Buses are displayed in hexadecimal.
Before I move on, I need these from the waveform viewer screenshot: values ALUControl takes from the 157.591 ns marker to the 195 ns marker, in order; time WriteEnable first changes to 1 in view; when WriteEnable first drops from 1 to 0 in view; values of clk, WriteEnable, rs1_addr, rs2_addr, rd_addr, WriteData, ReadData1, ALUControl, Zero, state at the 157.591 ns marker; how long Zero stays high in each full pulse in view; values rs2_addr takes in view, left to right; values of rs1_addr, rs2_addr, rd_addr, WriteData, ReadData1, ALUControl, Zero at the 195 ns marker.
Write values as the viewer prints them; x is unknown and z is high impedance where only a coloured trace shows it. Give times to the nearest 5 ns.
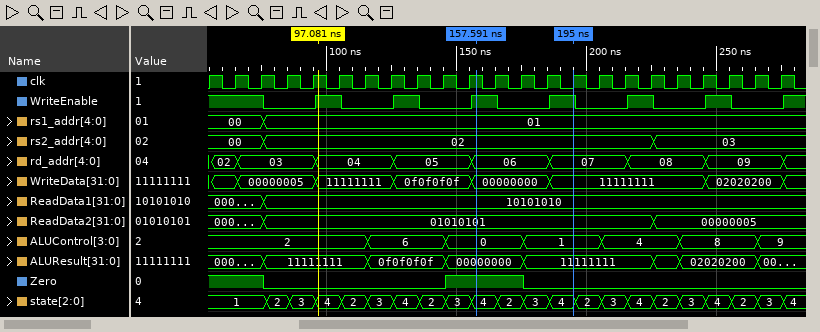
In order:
0, 1
95 ns
75 ns
clk=1, WriteEnable=1, rs1_addr=01, rs2_addr=02, rd_addr=06, WriteData=00000000, ReadData1=10101010, ALUControl=0, Zero=1, state=4
30 ns
00, 02, 03
rs1_addr=01, rs2_addr=02, rd_addr=07, WriteData=11111111, ReadData1=10101010, ALUControl=1, Zero=0
